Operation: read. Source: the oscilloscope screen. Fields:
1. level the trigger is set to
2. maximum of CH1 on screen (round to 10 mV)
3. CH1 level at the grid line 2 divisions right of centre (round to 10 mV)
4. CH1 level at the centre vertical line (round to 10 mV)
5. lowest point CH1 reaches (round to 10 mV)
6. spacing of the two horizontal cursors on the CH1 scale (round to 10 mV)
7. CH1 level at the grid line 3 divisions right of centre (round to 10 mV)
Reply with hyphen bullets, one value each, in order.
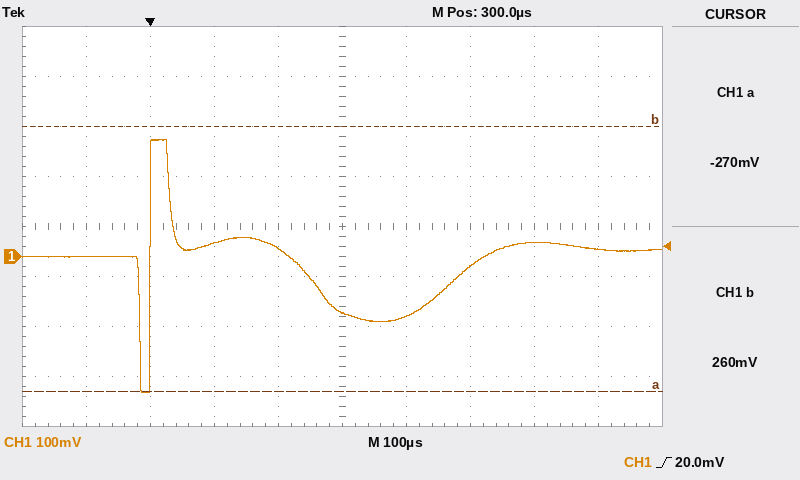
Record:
- 20.0 mV
- 230 mV
- -20 mV
- -110 mV
- -270 mV
- 530 mV
- 30 mV
